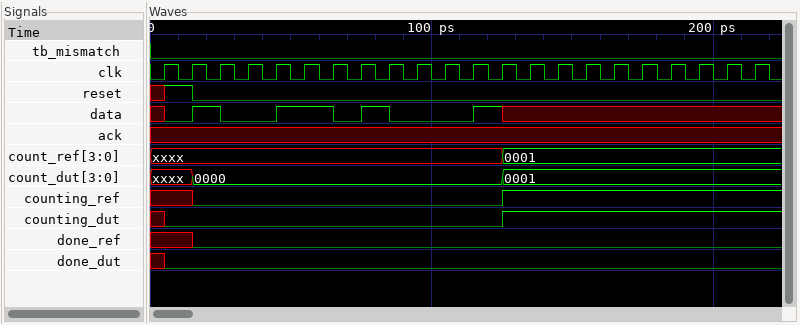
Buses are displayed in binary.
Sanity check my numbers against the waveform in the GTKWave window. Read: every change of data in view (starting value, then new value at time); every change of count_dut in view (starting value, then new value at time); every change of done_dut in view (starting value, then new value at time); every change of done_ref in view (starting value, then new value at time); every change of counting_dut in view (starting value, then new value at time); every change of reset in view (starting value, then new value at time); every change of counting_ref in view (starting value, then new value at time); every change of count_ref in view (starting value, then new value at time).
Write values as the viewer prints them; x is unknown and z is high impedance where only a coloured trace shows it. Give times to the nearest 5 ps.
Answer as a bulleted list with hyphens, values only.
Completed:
- x, 0 at 5 ps, 1 at 15 ps, 0 at 25 ps, 1 at 45 ps, 0 at 65 ps, 1 at 75 ps, 0 at 85 ps, 1 at 115 ps, x at 125 ps
- xxxx, 0000 at 15 ps, 0001 at 125 ps
- x, 0 at 5 ps
- x, 0 at 15 ps
- x, 0 at 5 ps, 1 at 125 ps
- x, 1 at 5 ps, 0 at 15 ps
- x, 0 at 15 ps, 1 at 125 ps
- xxxx, 0001 at 125 ps
